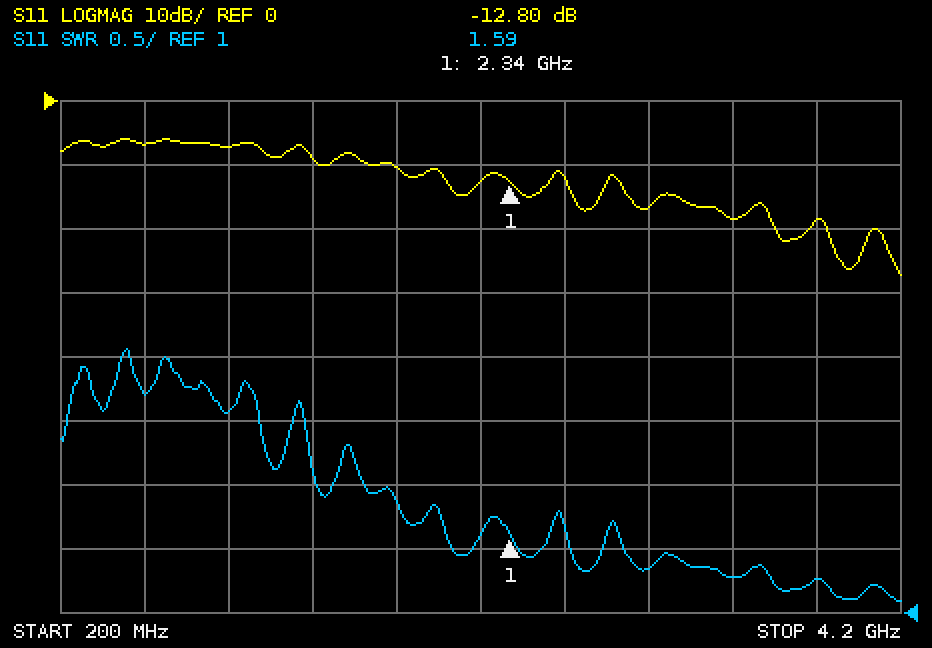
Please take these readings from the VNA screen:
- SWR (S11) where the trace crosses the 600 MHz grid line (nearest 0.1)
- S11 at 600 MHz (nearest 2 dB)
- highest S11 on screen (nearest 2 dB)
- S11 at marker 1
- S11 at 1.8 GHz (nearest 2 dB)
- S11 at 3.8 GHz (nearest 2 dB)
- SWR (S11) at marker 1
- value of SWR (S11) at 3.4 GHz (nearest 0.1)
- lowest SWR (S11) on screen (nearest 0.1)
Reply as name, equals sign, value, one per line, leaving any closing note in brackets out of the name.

SWR (S11) where the trace crosses the 600 MHz grid line = 2.7
S11 at 600 MHz = -6 dB
highest S11 on screen = -6 dB
S11 at marker 1 = -12.80 dB
S11 at 1.8 GHz = -10 dB
S11 at 3.8 GHz = -18 dB
SWR (S11) at marker 1 = 1.59
value of SWR (S11) at 3.4 GHz = 1.3
lowest SWR (S11) on screen = 1.1
